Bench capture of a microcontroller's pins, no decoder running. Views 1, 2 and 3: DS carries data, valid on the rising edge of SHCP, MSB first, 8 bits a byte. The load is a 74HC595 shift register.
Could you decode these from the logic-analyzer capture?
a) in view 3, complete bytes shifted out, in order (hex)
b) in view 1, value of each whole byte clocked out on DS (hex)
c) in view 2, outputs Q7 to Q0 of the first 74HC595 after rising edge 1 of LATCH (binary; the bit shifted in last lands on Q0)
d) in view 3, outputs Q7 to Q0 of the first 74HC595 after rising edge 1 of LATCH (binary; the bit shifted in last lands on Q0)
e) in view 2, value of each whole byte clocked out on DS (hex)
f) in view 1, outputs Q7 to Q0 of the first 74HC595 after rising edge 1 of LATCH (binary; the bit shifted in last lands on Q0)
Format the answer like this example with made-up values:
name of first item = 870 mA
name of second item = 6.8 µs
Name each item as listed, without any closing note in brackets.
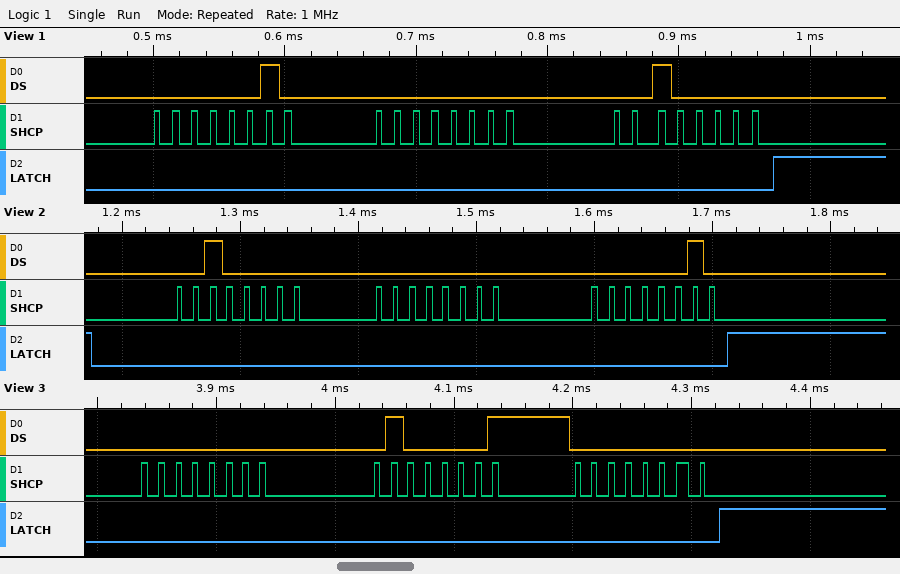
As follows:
in view 3, complete bytes shifted out, in order = 00 41 00
in view 1, value of each whole byte clocked out on DS = 02 00 20
in view 2, outputs Q7 to Q0 of the first 74HC595 after rising edge 1 of LATCH = 00000010
in view 3, outputs Q7 to Q0 of the first 74HC595 after rising edge 1 of LATCH = 00000000
in view 2, value of each whole byte clocked out on DS = 20 00 02
in view 1, outputs Q7 to Q0 of the first 74HC595 after rising edge 1 of LATCH = 00100000
